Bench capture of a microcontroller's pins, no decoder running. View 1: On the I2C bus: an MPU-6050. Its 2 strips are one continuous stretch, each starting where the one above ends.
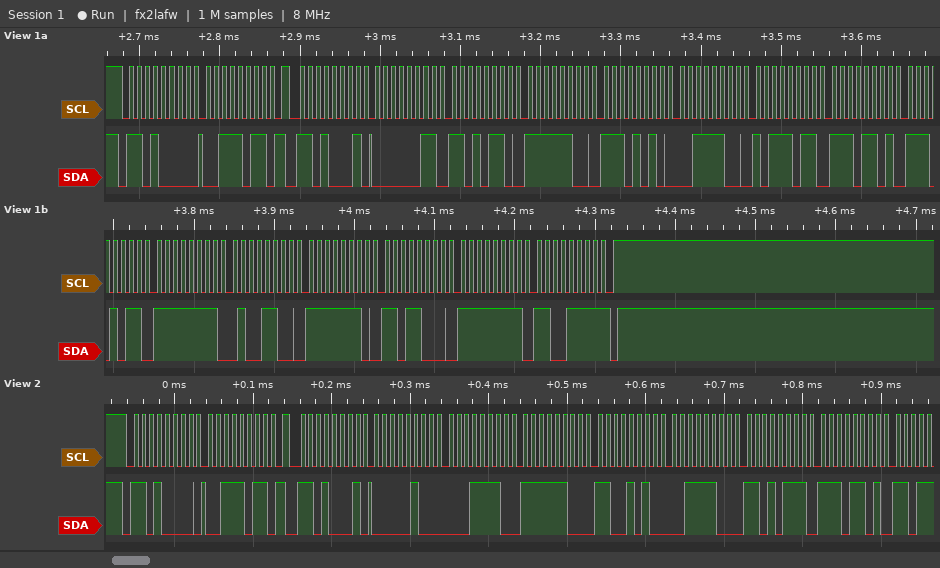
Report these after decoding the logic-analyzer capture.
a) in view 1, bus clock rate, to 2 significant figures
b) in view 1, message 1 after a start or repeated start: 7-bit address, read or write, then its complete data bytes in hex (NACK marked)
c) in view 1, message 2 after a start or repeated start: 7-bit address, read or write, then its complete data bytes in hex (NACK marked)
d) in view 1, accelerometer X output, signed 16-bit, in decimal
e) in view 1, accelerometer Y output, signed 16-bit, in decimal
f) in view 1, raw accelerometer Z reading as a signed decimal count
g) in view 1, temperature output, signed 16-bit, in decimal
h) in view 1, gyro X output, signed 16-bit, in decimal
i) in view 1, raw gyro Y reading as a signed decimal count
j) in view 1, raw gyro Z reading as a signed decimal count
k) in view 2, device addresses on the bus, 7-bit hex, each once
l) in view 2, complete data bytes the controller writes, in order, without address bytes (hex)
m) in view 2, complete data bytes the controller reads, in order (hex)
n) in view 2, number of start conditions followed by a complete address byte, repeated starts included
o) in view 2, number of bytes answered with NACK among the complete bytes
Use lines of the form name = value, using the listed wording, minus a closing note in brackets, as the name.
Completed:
in view 1, bus clock rate, to 2 significant figures = 100 kHz
in view 1, message 1 after a start or repeated start: 7-bit address, read or write, then its complete data bytes in hex = 0x68 write: 3B
in view 1, message 2 after a start or repeated start: 7-bit address, read or write, then its complete data bytes in hex = 0x68 read: 03 D6 FC EA 3C BB ED EB FF 4C FE D8 FF CF NACK
in view 1, accelerometer X output, signed 16-bit, in decimal = 982
in view 1, accelerometer Y output, signed 16-bit, in decimal = -790
in view 1, raw accelerometer Z reading as a signed decimal count = 15547
in view 1, temperature output, signed 16-bit, in decimal = -4629
in view 1, gyro X output, signed 16-bit, in decimal = -180
in view 1, raw gyro Y reading as a signed decimal count = -296
in view 1, raw gyro Z reading as a signed decimal count = -49
in view 2, device addresses on the bus, 7-bit hex, each once = 0x68
in view 2, complete data bytes the controller writes, in order, without address bytes = 3B
in view 2, complete data bytes the controller reads, in order = 04 1E FC CA 3C D7 ED
in view 2, number of start conditions followed by a complete address byte, repeated starts included = 2
in view 2, number of bytes answered with NACK among the complete bytes = 0
